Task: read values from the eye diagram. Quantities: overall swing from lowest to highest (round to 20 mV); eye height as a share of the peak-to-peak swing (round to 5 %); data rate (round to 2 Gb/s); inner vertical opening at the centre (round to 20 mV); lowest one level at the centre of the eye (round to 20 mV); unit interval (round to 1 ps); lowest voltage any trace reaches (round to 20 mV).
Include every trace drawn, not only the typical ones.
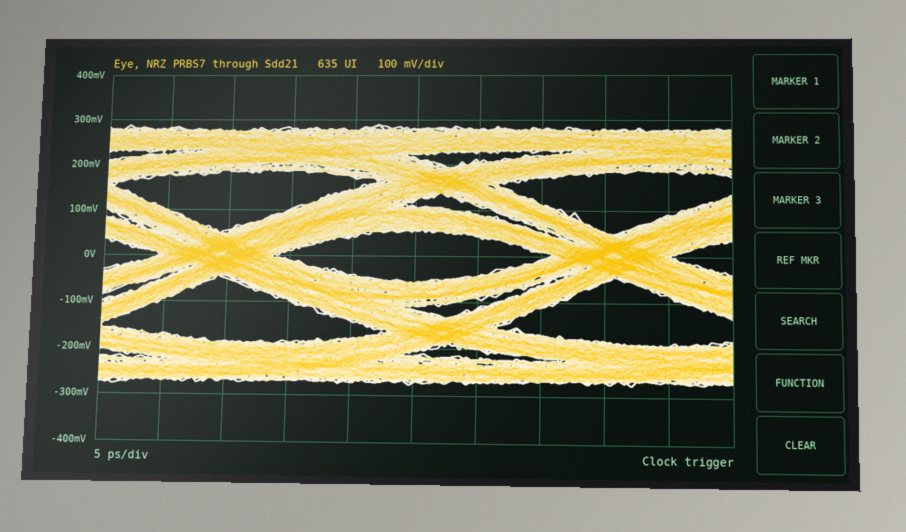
560 mV
20 %
32 Gb/s
120 mV
60 mV
31 ps
-280 mV
